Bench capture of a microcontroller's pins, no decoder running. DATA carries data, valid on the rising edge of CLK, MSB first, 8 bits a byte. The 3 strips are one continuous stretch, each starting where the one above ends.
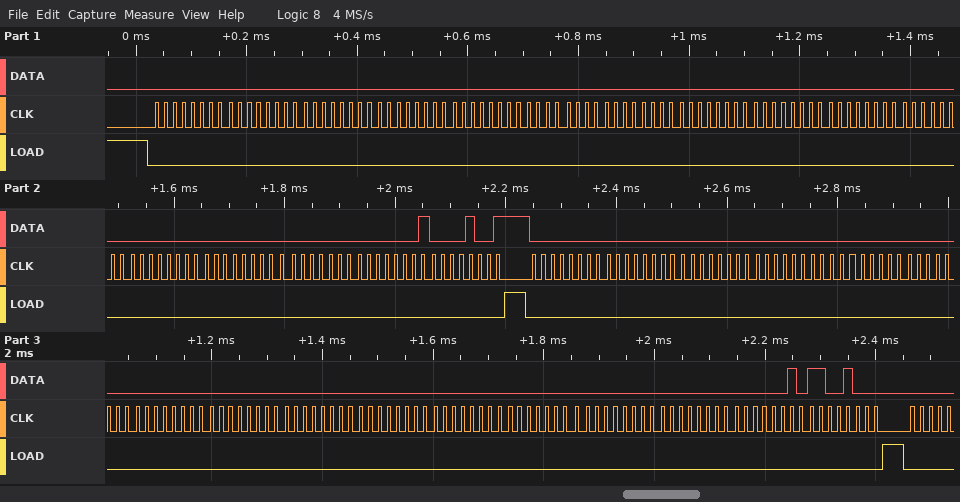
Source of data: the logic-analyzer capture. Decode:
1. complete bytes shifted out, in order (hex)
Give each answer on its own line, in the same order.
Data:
0x00 0x00 0x00 0x00 0x00 0x00 0x00 0x00 0x00 0x00 0x00 0x00 0x00 0x00 0x01 0x09 0x00 0x00 0x00 0x00 0x00 0x00 0x00 0x00 0x00 0x00 0x00 0x00 0x00 0x00 0x02 0xC8
